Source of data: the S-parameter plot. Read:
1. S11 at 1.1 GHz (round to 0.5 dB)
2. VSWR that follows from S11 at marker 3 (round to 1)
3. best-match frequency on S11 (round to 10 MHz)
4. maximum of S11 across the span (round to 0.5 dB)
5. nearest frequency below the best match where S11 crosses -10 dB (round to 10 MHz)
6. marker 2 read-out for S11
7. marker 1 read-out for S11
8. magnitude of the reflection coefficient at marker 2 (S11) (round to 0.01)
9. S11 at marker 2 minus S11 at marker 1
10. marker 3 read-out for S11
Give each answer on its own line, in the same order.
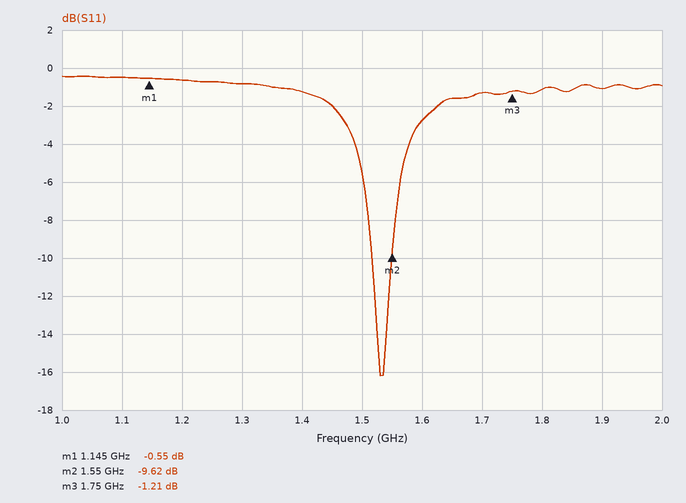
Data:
-0.5 dB
14
1.53 GHz
-0.5 dB
1.52 GHz
-9.62 dB
-0.55 dB
0.33
-9.07 dB
-1.21 dB
